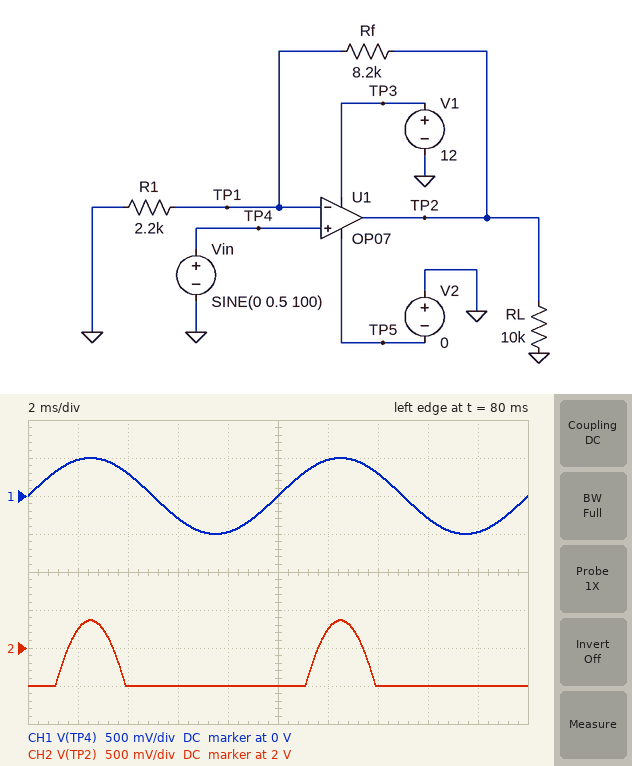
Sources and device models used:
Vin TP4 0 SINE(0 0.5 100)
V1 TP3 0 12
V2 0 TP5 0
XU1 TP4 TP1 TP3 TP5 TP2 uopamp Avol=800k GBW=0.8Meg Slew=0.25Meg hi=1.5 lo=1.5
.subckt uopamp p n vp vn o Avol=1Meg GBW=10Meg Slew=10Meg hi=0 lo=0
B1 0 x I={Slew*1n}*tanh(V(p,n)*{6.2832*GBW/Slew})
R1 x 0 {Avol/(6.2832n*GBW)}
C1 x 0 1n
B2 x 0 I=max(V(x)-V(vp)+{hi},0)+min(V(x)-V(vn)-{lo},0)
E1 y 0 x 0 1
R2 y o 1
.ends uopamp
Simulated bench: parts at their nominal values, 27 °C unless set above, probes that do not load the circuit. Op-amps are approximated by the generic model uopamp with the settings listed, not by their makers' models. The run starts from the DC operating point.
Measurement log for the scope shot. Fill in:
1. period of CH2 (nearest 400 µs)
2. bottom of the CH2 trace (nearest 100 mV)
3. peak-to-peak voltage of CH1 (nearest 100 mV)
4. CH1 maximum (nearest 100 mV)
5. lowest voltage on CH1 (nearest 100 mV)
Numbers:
10.0 ms
1.5 V
1.0 V
500 mV
-500 mV
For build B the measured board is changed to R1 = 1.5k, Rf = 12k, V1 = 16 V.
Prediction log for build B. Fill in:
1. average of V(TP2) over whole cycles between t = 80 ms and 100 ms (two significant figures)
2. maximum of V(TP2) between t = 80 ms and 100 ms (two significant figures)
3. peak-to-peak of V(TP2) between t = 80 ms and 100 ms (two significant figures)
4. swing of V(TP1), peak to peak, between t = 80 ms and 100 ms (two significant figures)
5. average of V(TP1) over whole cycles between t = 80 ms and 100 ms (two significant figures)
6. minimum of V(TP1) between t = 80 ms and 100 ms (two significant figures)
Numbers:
2.3 V
4.5 V
3.0 V
330 mV
250 mV
170 mV
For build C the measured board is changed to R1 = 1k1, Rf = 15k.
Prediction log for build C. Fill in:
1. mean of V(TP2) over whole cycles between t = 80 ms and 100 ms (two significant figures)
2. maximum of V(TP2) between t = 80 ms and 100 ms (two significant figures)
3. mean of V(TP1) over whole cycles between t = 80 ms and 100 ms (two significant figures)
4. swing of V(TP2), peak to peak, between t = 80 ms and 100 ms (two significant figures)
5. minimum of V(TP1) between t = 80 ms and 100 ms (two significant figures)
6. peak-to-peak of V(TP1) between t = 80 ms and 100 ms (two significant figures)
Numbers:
3.1 V
7.3 V
210 mV
5.8 V
100 mV
400 mV
